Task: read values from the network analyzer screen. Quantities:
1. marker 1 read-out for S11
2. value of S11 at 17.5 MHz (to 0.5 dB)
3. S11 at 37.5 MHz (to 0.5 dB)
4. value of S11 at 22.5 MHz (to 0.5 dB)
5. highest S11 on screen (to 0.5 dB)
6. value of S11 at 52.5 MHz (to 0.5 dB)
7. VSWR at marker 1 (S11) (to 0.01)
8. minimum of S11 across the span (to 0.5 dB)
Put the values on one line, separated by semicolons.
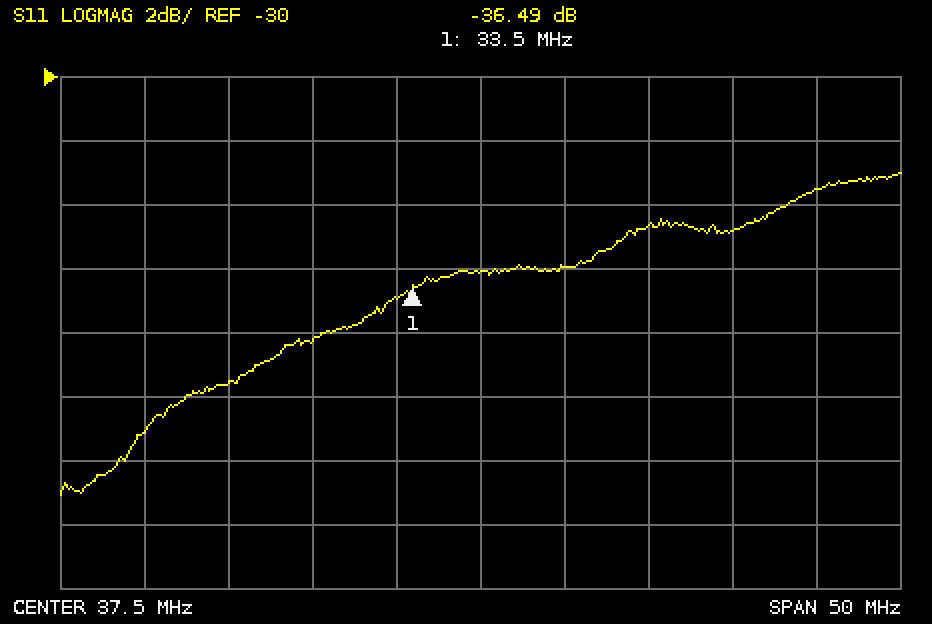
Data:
-36.49 dB; -41.0 dB; -36.0 dB; -39.5 dB; -33.0 dB; -35.0 dB; 1.03; -43.0 dB
